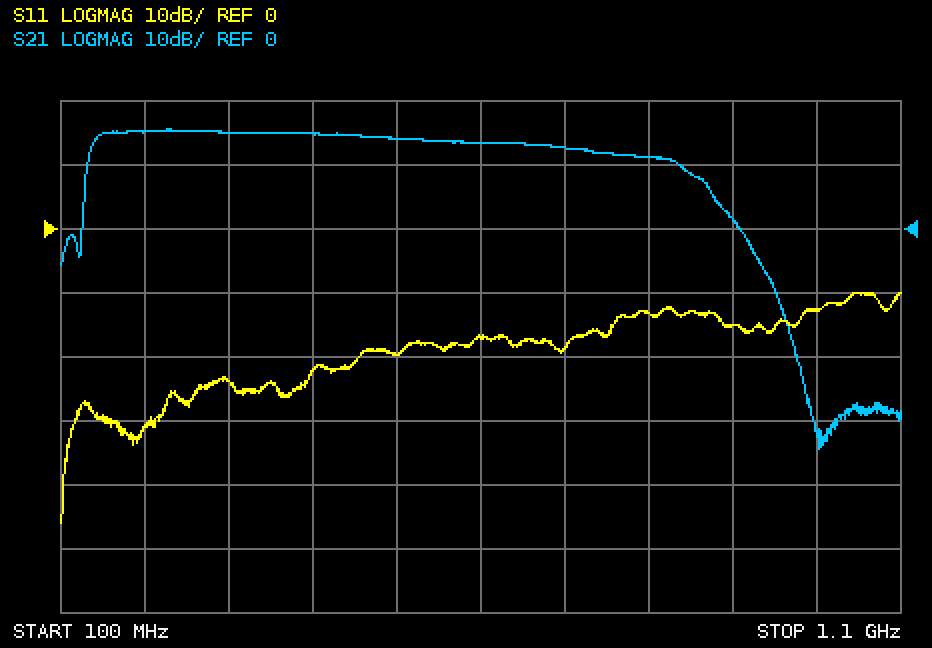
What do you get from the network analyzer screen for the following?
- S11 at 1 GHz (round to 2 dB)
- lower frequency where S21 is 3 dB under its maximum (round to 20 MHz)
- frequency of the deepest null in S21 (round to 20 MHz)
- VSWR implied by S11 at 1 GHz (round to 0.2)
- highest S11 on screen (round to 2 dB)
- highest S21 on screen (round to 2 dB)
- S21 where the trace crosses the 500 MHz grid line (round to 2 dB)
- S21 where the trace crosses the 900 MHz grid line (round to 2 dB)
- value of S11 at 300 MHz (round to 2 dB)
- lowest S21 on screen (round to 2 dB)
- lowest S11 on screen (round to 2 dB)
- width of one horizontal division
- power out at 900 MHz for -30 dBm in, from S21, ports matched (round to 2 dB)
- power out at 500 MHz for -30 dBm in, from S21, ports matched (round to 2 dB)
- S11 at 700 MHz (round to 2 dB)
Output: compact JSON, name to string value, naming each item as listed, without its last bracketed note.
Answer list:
{"S11 at 1 GHz": "-12 dB", "lower frequency where S21 is 3 dB under its maximum": "140 MHz", "frequency of the deepest null in S21": "1.00 GHz", "VSWR implied by S11 at 1 GHz": "1.6", "highest S11 on screen": "-10 dB", "highest S21 on screen": "16 dB", "S21 where the trace crosses the 500 MHz grid line": "14 dB", "S21 where the trace crosses the 900 MHz grid line": "2 dB", "value of S11 at 300 MHz": "-24 dB", "lowest S21 on screen": "-34 dB", "lowest S11 on screen": "-46 dB", "width of one horizontal division": "100 MHz", "power out at 900 MHz for -30 dBm in, from S21, ports matched": "-28 dBm", "power out at 500 MHz for -30 dBm in, from S21, ports matched": "-16 dBm", "S11 at 700 MHz": "-18 dB"}
